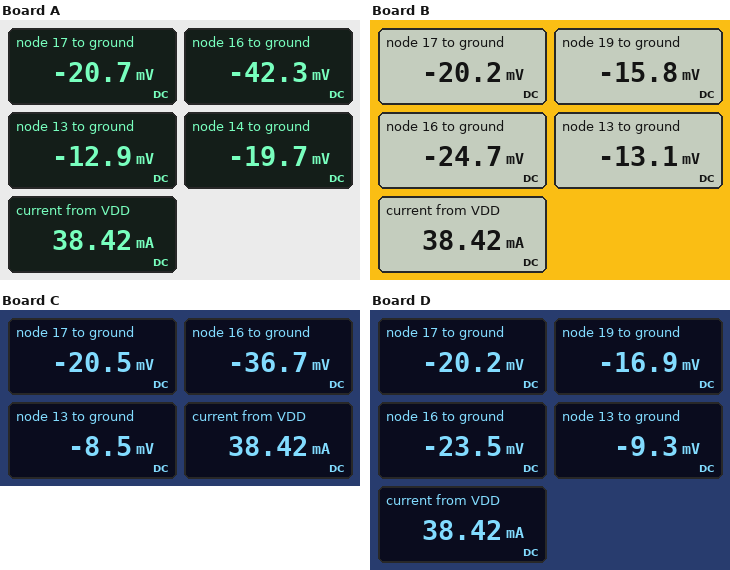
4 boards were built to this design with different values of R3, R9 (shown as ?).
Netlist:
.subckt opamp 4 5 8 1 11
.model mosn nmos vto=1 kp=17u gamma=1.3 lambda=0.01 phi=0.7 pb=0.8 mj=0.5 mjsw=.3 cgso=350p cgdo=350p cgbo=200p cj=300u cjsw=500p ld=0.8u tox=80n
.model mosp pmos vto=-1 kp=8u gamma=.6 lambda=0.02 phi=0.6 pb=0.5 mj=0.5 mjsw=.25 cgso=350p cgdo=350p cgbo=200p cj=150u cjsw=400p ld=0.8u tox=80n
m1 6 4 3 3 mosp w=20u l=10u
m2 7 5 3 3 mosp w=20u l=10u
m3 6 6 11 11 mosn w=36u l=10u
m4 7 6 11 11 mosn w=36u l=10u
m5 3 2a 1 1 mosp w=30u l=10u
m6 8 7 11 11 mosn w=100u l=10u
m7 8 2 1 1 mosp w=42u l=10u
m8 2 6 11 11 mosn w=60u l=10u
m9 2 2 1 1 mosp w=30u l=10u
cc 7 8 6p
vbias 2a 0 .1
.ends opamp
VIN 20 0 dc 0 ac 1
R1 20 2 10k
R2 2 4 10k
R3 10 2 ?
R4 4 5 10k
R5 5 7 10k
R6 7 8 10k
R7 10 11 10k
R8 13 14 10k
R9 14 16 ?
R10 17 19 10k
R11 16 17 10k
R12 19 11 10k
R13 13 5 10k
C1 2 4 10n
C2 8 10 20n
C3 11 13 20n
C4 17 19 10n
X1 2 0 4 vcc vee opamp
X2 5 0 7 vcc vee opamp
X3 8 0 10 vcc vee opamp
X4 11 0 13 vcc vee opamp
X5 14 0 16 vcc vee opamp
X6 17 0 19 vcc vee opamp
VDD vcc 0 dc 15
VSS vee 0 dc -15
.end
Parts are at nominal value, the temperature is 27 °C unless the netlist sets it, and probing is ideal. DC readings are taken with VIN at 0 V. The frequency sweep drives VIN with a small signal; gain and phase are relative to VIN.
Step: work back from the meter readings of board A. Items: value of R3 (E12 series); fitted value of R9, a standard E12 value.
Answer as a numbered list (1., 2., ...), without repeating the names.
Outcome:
1. 18 kΩ
2. 33 kΩ
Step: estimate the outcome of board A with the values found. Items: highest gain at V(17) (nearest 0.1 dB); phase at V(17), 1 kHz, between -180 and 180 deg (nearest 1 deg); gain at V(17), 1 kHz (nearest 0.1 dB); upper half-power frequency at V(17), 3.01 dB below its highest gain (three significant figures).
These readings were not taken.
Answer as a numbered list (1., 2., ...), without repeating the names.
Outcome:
1. -31.7 dB
2. 77 deg
3. -35.6 dB
4. 823 Hz
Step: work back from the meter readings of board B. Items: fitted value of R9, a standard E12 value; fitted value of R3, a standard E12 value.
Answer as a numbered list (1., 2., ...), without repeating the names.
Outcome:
1. 6.8 kΩ
2. 3.9 kΩ
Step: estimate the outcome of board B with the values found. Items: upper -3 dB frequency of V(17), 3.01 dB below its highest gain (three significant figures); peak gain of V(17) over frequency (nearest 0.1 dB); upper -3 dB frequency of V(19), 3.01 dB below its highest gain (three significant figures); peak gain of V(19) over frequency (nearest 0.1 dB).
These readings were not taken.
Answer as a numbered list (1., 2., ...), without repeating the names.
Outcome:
1. 1.28 kHz
2. -45.3 dB
3. 1.20 kHz
4. -13.3 dB
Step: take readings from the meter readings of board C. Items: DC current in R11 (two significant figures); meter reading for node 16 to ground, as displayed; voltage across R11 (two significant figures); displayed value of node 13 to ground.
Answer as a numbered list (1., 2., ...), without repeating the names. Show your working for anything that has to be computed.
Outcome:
1. (-20.5 mV - (-36.7 mV)) / 10 kΩ = 1.6 µA
2. -36.7 mV
3. -20.5 mV - (-36.7 mV) = 16 mV
4. -8.5 mV
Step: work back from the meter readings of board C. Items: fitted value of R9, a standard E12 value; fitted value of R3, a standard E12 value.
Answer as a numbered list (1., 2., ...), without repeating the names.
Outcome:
1. 15 kΩ
2. 22 kΩ
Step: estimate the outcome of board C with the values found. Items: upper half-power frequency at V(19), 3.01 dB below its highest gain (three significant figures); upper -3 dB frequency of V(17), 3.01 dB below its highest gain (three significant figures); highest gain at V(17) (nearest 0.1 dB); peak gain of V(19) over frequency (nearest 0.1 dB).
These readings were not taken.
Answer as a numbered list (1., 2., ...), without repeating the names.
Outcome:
1. 1.16 kHz
2. 1.20 kHz
3. -34.2 dB
4. -2.1 dB
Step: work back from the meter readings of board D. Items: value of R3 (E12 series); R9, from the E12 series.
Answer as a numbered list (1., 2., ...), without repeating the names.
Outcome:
1. 4.7 kΩ
2. 3.3 kΩ
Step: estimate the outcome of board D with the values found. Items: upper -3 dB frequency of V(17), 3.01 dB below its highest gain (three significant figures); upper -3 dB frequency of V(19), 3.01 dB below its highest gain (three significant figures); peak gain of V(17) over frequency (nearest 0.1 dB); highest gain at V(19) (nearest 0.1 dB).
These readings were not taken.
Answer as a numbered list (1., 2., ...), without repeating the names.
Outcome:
1. 827 Hz
2. 796 Hz
3. -47.8 dB
4. -15.9 dB
